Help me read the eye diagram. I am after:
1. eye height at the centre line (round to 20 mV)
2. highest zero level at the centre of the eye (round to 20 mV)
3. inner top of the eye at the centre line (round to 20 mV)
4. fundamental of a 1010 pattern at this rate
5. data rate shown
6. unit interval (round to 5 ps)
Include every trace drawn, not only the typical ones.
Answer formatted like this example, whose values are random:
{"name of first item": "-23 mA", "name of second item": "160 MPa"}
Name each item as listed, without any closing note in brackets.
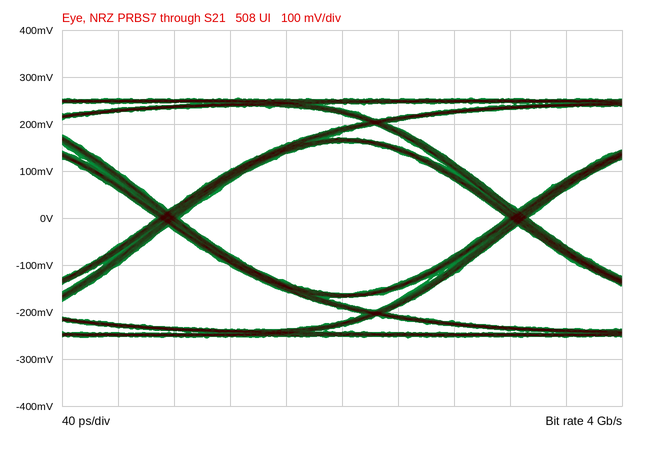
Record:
{"eye height at the centre line": "320 mV", "highest zero level at the centre of the eye": "-160 mV", "inner top of the eye at the centre line": "160 mV", "fundamental of a 1010 pattern at this rate": "2 GHz", "data rate shown": "4 Gb/s", "unit interval": "250 ps"}
